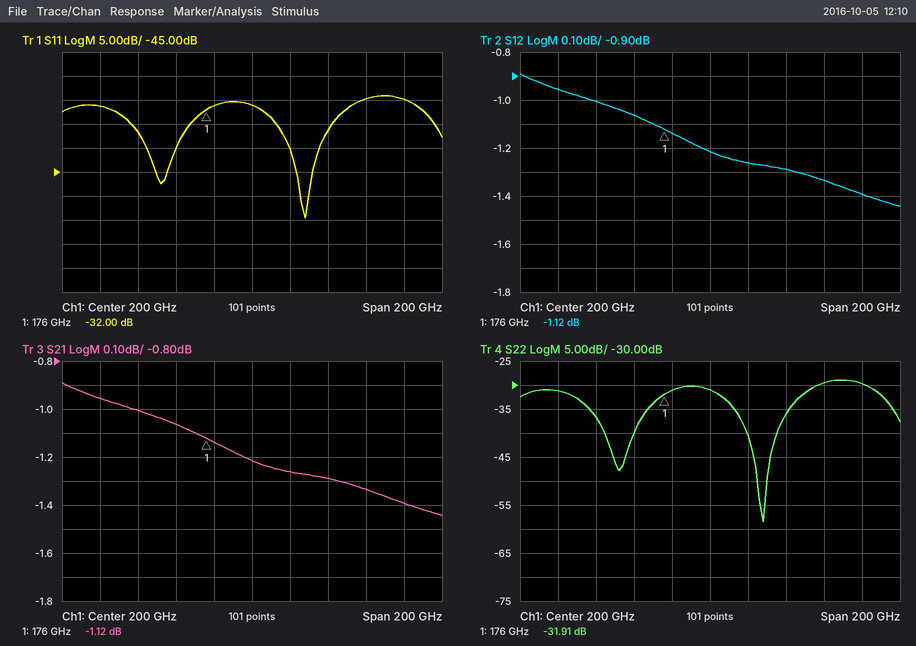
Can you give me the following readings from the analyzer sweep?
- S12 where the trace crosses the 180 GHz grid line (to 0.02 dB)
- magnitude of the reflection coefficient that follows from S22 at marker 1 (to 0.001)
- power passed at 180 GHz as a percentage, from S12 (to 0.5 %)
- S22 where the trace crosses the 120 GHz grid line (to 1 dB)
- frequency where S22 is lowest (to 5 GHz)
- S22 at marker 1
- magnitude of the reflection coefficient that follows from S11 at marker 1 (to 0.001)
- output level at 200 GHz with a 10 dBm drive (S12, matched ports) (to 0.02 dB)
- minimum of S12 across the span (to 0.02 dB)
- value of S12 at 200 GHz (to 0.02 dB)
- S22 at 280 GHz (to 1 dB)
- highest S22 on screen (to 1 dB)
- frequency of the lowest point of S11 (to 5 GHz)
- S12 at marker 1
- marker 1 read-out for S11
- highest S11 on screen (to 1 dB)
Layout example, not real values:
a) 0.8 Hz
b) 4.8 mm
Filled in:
a) -1.14 dB
b) 0.025
c) 77.0 %
d) -31 dB
e) 230 GHz
f) -31.91 dB
g) 0.025
h) 8.78 dBm
i) -1.44 dB
j) -1.22 dB
k) -30 dB
l) -29 dB
m) 230 GHz
n) -1.12 dB
o) -32.00 dB
p) -29 dB
